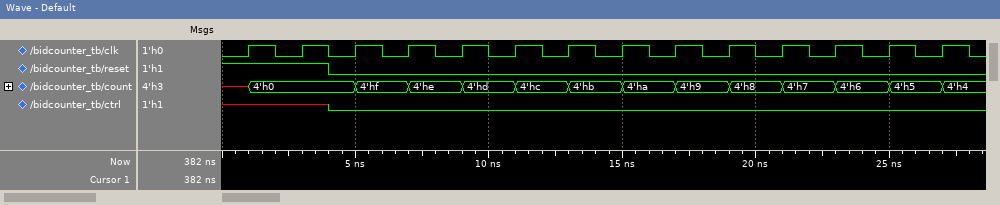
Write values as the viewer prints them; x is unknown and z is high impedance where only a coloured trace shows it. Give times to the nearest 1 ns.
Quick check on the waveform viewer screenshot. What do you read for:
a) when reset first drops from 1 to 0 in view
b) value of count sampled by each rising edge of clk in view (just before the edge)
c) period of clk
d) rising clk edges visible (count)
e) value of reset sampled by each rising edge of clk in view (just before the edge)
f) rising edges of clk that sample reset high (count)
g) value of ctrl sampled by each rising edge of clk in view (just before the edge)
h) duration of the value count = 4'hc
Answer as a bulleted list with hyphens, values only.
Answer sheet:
- 4 ns
- x, 4'h0, 4'h0, 4'hf, 4'he, 4'hd, 4'hc, 4'hb, 4'ha, 4'h9, 4'h8, 4'h7, 4'h6, 4'h5
- 2 ns
- 14
- 1 1 0 0 0 0 0 0 0 0 0 0 0 0
- 2
- x x 0 0 0 0 0 0 0 0 0 0 0 0
- 2 ns
